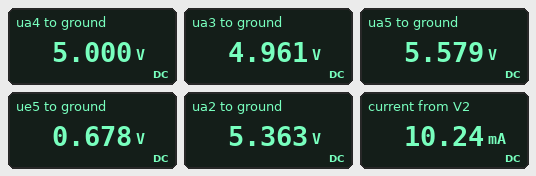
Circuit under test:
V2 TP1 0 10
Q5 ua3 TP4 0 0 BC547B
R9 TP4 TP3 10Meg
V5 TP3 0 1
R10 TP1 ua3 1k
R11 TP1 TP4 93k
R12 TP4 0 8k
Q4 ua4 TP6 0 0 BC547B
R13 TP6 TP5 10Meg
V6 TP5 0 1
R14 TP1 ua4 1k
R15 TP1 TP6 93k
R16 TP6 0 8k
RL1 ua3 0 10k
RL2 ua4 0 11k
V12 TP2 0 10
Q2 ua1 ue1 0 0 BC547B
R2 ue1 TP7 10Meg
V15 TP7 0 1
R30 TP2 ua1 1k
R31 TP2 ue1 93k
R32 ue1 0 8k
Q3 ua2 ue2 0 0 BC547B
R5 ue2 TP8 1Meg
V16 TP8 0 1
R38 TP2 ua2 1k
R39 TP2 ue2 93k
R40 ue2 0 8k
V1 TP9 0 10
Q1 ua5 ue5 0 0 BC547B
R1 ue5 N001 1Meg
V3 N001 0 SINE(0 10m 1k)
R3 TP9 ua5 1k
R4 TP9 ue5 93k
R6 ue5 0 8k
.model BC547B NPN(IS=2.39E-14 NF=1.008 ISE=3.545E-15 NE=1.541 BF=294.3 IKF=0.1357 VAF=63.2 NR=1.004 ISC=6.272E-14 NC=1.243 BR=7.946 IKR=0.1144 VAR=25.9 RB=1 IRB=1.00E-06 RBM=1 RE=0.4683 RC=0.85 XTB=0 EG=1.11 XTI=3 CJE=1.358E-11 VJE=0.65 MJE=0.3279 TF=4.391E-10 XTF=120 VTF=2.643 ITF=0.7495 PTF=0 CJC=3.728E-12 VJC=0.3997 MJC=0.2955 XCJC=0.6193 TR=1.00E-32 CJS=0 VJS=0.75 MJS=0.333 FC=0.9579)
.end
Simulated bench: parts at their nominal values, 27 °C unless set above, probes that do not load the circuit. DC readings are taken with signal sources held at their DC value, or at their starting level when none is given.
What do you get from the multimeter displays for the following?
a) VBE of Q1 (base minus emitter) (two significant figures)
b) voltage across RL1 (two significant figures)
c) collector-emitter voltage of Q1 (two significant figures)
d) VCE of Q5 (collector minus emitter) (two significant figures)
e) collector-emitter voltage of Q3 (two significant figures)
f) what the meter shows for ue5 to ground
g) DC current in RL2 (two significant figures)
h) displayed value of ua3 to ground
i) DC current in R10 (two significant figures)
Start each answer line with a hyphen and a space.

- 680 mV
- 5.0 V
- 5.6 V
- 5.0 V
- 5.4 V
- 0.678 V
- 450 µA
- 4.961 V
- 5.0 mA
